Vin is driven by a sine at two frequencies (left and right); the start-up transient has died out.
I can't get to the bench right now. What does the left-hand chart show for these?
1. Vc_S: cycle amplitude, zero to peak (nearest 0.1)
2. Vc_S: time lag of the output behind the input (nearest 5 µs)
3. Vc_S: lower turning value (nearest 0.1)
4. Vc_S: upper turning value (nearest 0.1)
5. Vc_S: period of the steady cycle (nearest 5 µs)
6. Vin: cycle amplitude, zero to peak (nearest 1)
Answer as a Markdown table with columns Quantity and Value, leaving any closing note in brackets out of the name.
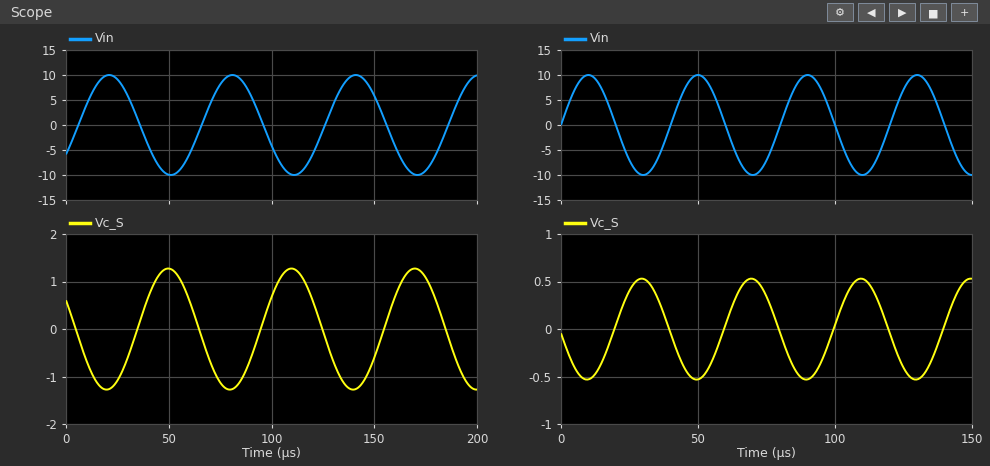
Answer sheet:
| Quantity | Value |
|---|---|
| Vc_S: cycle amplitude, zero to peak | 1.3 |
| Vc_S: time lag of the output behind the input | 30 µs |
| Vc_S: lower turning value | -1.3 |
| Vc_S: upper turning value | 1.3 |
| Vc_S: period of the steady cycle | 60 µs |
| Vin: cycle amplitude, zero to peak | 10 |
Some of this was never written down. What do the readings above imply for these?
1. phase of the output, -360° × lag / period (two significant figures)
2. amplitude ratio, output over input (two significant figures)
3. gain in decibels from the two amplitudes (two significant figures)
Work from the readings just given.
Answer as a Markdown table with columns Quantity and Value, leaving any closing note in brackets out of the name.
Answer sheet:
| Quantity | Value |
|---|---|
| phase of the output, -360° × lag / period | -180° |
| amplitude ratio, output over input | 0.13 |
| gain in decibels from the two amplitudes | -18 dB |
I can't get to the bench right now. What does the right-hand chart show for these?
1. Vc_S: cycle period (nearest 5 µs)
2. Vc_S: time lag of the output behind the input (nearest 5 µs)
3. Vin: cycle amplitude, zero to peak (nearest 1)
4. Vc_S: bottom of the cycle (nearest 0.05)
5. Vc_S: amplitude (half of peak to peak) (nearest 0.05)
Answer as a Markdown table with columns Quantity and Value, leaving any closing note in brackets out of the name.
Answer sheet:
| Quantity | Value |
|---|---|
| Vc_S: cycle period | 40 µs |
| Vc_S: time lag of the output behind the input | 20 µs |
| Vin: cycle amplitude, zero to peak | 10 |
| Vc_S: bottom of the cycle | -0.55 |
| Vc_S: amplitude (half of peak to peak) | 0.55 |
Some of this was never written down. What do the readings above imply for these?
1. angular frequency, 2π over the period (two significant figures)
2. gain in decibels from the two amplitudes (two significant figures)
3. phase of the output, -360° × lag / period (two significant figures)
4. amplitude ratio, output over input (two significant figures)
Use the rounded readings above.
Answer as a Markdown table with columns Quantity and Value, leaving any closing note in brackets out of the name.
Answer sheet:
| Quantity | Value |
|---|---|
| angular frequency, 2π over the period | 0.16 rad/µs |
| gain in decibels from the two amplitudes | -25 dB |
| phase of the output, -360° × lag / period | -180° |
| amplitude ratio, output over input | 0.055 |
